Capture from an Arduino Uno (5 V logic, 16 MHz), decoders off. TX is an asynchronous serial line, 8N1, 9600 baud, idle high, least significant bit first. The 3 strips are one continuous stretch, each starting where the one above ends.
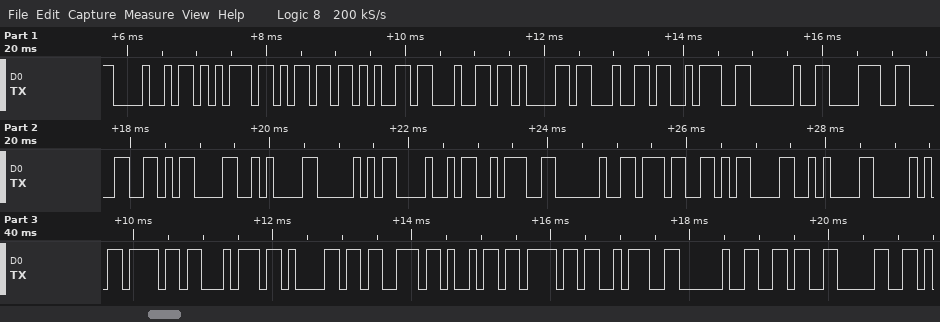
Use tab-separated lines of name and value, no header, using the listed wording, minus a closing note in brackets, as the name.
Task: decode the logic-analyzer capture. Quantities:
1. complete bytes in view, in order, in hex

complete bytes in view, in order, in hex	48 75 6D 65 64 61 64 3A 20 38 30 0D 0A 50 48 3A 20 37 0D 0A 50 6F 74 61 73 69 6F 3A 20 36 30
